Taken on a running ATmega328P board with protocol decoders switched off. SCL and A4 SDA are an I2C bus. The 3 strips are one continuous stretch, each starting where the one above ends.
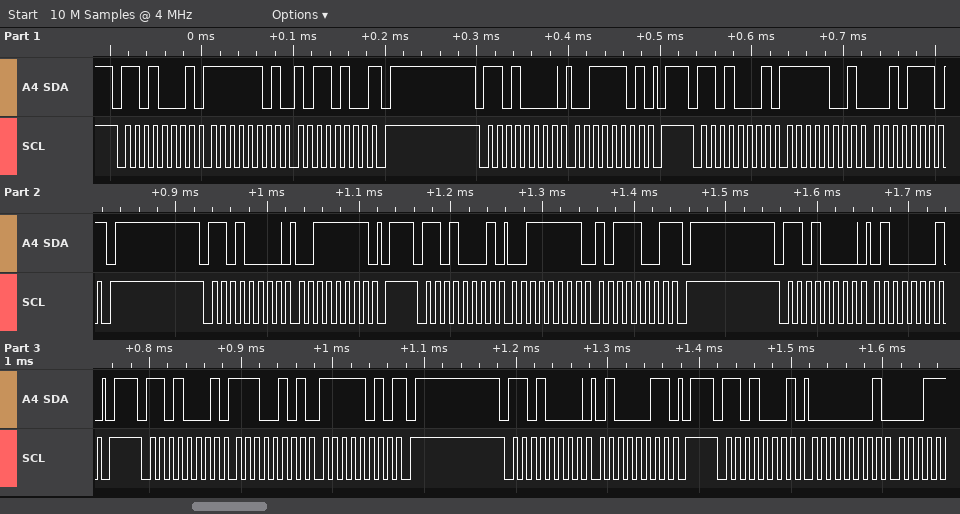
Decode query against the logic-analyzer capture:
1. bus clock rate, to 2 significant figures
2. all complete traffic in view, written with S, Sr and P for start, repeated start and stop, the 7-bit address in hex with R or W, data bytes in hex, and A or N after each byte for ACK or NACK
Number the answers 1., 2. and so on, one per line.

1. 100 kHz
2. S 68R A FD A B4 N P S 68W A 3D A P S 68R A F9 A 2E N P S 68W A 3F A P S 68R A 3F A B9 N P S 68W A 41 A P S 68R A E5 A FA N P S 68W A 43 A P S 68R A 01 A
